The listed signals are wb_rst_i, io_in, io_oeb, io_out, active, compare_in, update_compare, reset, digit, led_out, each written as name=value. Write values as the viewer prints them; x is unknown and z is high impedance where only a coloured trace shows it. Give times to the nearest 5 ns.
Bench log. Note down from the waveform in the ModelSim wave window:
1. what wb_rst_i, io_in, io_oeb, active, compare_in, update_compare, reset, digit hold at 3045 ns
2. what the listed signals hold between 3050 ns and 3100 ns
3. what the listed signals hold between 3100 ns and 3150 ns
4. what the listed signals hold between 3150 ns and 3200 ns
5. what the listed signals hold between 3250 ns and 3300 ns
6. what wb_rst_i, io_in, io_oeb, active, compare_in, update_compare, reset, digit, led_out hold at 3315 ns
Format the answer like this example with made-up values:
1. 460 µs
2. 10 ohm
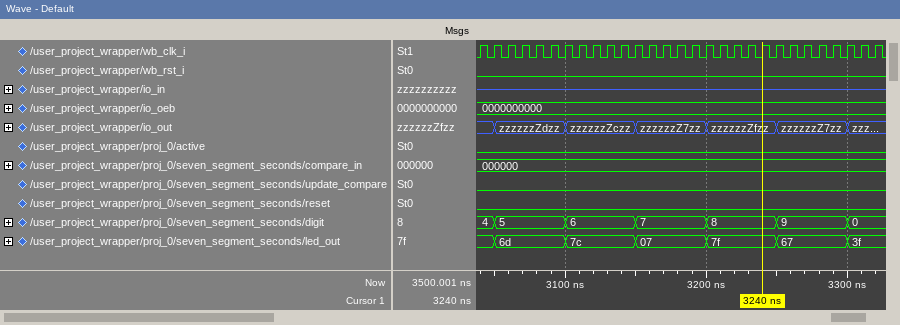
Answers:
1. wb_rst_i=0, io_in=z, io_oeb=0000000000, active=0, compare_in=000000, update_compare=0, reset=0, digit=4
2. wb_rst_i=0, io_in=z, io_oeb=0000000000, io_out=zzzzzzZdzz, active=0, compare_in=000000, update_compare=0, reset=0, digit=5, led_out=6d
3. wb_rst_i=0, io_in=z, io_oeb=0000000000, io_out=zzzzzzZczz, active=0, compare_in=000000, update_compare=0, reset=0, digit=6, led_out=7c
4. wb_rst_i=0, io_in=z, io_oeb=0000000000, io_out=zzzzzzZ7zz, active=0, compare_in=000000, update_compare=0, reset=0, digit=7, led_out=07
5. wb_rst_i=0, io_in=z, io_oeb=0000000000, io_out=zzzzzzZ7zz, active=0, compare_in=000000, update_compare=0, reset=0, digit=9, led_out=67
6. wb_rst_i=0, io_in=z, io_oeb=0000000000, active=0, compare_in=000000, update_compare=0, reset=0, digit=0, led_out=3f
